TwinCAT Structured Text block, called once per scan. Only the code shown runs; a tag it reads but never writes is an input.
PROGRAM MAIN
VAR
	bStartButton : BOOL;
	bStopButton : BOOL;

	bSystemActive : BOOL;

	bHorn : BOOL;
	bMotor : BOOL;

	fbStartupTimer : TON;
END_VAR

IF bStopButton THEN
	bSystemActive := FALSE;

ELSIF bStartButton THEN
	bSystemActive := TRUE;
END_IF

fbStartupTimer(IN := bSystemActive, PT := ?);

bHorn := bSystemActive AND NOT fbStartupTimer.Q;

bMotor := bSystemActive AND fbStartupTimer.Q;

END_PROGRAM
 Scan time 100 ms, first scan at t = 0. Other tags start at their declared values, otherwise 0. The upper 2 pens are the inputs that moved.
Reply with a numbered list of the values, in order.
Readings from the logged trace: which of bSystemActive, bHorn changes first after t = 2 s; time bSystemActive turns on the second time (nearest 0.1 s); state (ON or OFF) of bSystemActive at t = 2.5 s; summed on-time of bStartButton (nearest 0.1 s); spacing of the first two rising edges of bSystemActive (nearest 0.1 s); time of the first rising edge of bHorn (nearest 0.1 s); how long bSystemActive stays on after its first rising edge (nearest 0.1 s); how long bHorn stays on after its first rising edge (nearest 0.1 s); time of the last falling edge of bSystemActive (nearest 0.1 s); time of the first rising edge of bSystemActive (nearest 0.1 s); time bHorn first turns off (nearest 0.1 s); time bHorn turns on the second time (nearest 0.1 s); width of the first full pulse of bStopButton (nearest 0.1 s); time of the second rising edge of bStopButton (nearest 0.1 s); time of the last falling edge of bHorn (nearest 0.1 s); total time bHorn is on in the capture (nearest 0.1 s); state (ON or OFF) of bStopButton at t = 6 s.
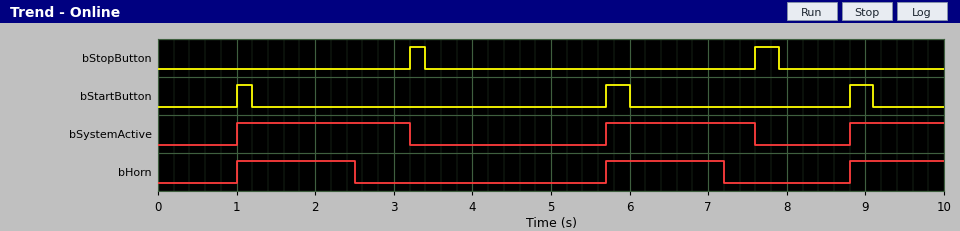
1. bHorn
2. 5.7 s
3. ON
4. 0.8 s
5. 4.7 s
6. 1.0 s
7. 2.2 s
8. 1.5 s
9. 7.6 s
10. 1.0 s
11. 2.5 s
12. 5.7 s
13. 0.2 s
14. 7.6 s
15. 7.2 s
16. 4.2 s
17. OFF
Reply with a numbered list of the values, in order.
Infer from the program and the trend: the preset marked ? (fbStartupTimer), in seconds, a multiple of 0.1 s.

1. 1.5 s
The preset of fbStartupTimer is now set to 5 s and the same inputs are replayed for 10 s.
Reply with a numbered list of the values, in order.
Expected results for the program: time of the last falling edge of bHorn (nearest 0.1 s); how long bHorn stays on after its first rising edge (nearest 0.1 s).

1. 7.6 s
2. 2.2 s
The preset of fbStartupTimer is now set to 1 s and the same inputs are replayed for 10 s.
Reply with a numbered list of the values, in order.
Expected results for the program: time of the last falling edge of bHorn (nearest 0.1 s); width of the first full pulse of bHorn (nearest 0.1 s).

1. 9.8 s
2. 1.0 s
